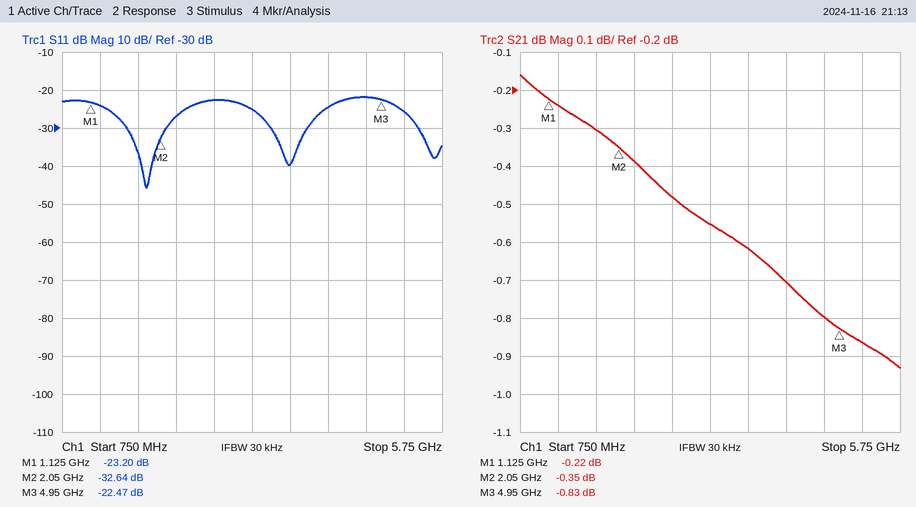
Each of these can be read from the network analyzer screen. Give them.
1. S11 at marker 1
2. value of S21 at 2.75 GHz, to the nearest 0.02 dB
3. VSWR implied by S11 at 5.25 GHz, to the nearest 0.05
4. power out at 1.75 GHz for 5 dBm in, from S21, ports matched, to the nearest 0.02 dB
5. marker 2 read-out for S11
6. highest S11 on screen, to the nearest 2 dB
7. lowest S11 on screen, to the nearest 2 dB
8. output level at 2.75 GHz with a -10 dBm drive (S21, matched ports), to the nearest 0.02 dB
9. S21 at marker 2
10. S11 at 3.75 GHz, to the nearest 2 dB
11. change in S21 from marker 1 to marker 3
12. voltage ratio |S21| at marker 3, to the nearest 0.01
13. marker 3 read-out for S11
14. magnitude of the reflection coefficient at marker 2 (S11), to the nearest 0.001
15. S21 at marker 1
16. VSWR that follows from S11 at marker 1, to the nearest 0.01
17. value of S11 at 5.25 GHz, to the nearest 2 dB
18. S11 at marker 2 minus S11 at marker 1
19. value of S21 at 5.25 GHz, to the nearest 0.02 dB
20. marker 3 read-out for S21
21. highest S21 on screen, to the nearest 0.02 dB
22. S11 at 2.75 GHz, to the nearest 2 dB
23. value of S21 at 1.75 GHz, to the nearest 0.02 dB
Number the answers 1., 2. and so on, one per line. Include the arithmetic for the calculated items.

1. -23.20 dB
2. -0.48 dB
3. |Γ| = 10^(-26/20) = 0.0501; VSWR = (1 + 0.0501)/(1 − 0.0501) ≈ 1.11, so 1.10 to the nearest 0.05
4. 5 dBm + (-0.30 dB) = 4.70 dBm
5. -32.64 dB
6. -22 dB
7. -46 dB
8. -10 dBm + (-0.48 dB) = -10.48 dBm
9. -0.35 dB
10. -40 dB
11. -0.83 − (-0.22) = -0.61 dB
12. 10^(-0.83/20) ≈ 0.91
13. -22.47 dB
14. 10^(-32.64/20) ≈ 0.023
15. -0.22 dB
16. (1 + 0.0692)/(1 − 0.0692) ≈ 1.15
17. -26 dB
18. -32.64 − (-23.2) = -9.44 dB
19. -0.86 dB
20. -0.83 dB
21. -0.16 dB
22. -22 dB
23. -0.30 dB
